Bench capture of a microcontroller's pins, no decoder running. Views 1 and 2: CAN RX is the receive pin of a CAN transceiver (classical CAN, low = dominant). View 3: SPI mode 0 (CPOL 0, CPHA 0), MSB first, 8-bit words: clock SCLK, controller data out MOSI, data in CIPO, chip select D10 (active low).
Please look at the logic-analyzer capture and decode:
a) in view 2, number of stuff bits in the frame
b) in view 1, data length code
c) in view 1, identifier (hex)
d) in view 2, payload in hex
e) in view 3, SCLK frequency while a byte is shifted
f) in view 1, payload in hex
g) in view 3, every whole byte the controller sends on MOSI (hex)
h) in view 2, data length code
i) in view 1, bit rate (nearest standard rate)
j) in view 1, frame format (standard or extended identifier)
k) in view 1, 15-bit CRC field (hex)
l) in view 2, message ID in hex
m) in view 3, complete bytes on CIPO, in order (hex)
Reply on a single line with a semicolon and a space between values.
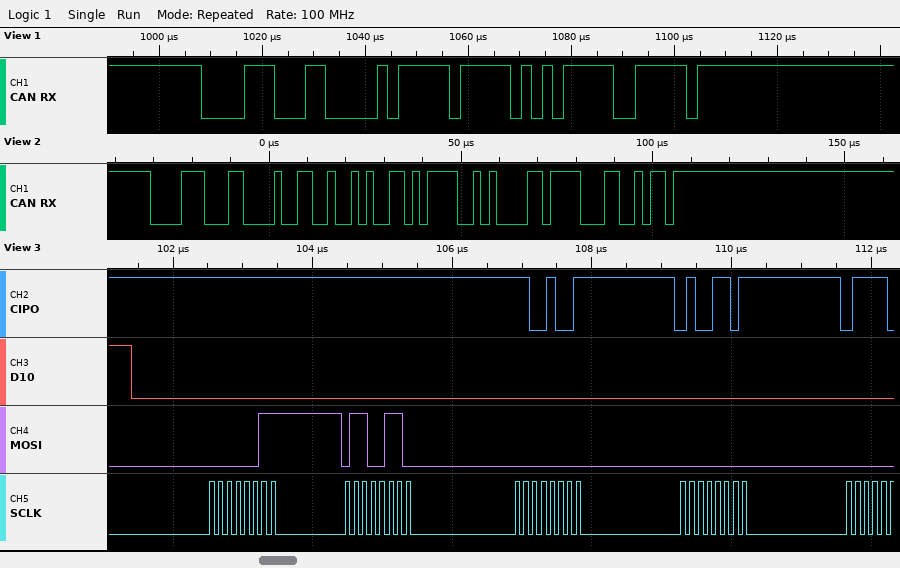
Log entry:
0; 1; 0x0E3; C9 4D 79 43; 8 MHz; FF; 03 66 00 00; 4; 500 kbit/s; standard; 0x6BEF; 0x0E3; FF FF C9 4D
